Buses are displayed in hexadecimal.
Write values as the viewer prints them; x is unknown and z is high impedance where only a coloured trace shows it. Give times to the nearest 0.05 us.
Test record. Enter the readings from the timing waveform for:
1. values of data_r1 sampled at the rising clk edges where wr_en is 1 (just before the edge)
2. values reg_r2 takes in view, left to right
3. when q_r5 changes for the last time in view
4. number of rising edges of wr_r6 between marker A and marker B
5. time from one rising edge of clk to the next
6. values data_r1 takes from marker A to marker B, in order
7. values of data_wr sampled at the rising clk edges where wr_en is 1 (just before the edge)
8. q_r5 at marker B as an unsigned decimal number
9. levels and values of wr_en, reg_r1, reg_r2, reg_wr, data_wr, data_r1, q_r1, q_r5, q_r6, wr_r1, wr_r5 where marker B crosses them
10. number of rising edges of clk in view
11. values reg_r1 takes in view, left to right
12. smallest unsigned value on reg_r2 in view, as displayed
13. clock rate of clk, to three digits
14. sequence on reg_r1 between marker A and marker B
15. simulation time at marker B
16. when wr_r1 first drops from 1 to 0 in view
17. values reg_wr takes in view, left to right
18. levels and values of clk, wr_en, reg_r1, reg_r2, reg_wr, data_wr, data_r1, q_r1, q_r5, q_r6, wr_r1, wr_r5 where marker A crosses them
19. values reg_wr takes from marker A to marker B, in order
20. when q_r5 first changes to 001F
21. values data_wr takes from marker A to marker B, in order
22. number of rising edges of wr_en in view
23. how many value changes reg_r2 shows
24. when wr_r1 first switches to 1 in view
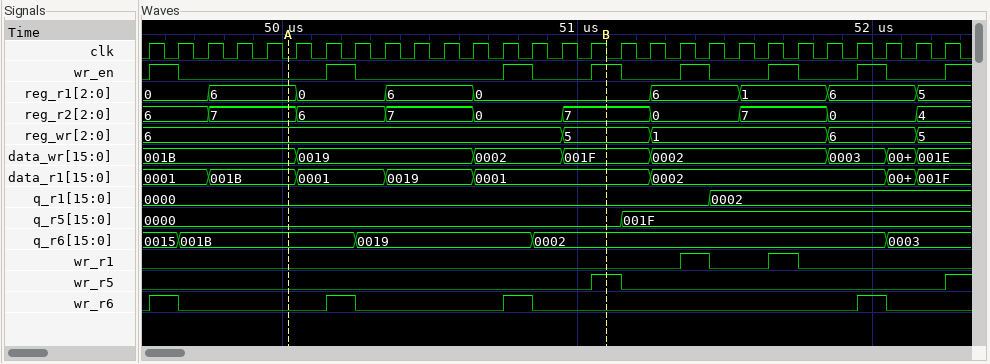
0001, 0001, 0001, 0001, 0002, 0002, 0002
6, 7, 6, 7, 0, 7, 0, 7, 0, 4
51.15 us
2
0.1 us
001B, 0001, 0019, 0001
001B, 0019, 0002, 001F, 0002, 0002, 0003
0
wr_en=1, reg_r1=0, reg_r2=7, reg_wr=5, data_wr=001F, data_r1=0001, q_r1=0000, q_r5=0000, q_r6=0002, wr_r1=0, wr_r5=1
28
0, 6, 0, 6, 0, 6, 1, 6, 5
0
10.0 MHz
6, 0, 6, 0
51.1 us
51.45 us
6, 5, 1, 6, 5
clk=0, wr_en=0, reg_r1=6, reg_r2=7, reg_wr=6, data_wr=001B, data_r1=001B, q_r1=0000, q_r5=0000, q_r6=001B, wr_r1=0, wr_r5=0
6, 5
51.15 us
001B, 0019, 0002, 001F
8
9
51.35 us
